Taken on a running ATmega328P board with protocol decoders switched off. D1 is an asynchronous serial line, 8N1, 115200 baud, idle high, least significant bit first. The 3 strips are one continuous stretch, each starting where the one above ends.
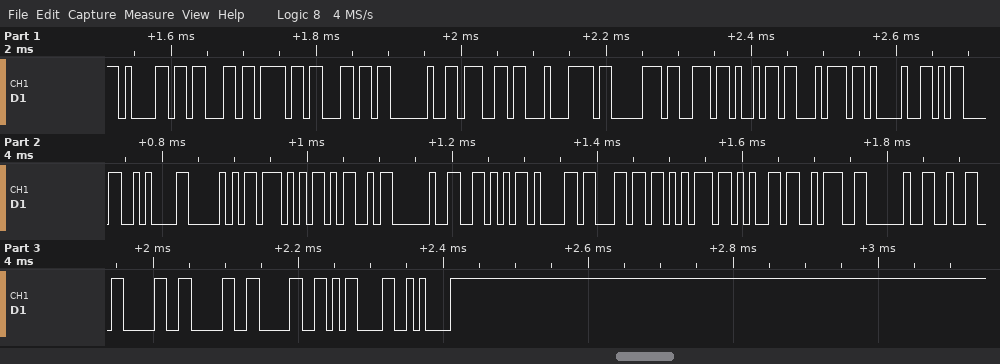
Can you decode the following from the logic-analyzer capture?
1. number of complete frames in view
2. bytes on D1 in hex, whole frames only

31
61 63 6F 6C 20 67 C4 83 73 69 74 21 0D 0A 50 57 4D 20 56 61 6C 75 65 3A 20 32 30 30 30 0D 0A
